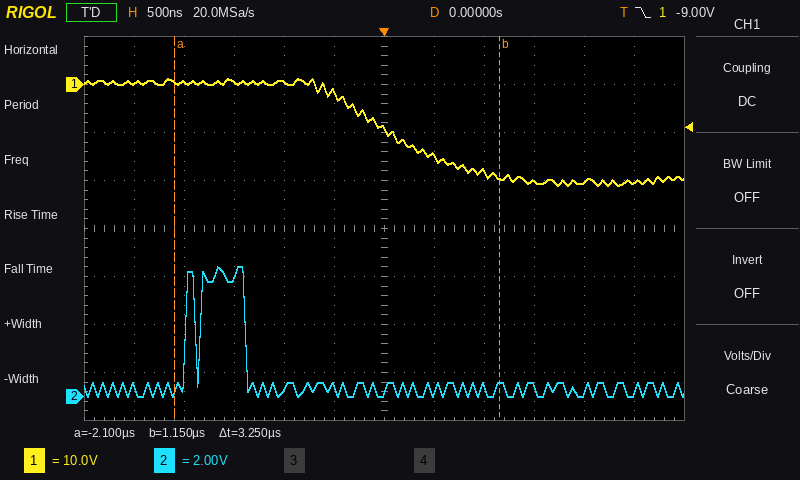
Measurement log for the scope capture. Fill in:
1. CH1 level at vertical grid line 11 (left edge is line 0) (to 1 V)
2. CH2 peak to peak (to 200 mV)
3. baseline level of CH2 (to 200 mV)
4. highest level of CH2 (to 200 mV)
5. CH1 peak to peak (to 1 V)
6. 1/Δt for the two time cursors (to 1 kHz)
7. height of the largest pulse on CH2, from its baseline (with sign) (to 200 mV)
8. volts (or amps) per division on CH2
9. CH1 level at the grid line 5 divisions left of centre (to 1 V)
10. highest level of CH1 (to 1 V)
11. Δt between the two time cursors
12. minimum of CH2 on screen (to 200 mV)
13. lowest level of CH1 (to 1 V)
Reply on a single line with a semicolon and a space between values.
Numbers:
-20 V; 5.4 V; 400 mV; 5.4 V; 22 V; 308 kHz; +5.0 V; 2 V; 0 V; 1 V; 3.25 µs; 0.0 V; -21 V
